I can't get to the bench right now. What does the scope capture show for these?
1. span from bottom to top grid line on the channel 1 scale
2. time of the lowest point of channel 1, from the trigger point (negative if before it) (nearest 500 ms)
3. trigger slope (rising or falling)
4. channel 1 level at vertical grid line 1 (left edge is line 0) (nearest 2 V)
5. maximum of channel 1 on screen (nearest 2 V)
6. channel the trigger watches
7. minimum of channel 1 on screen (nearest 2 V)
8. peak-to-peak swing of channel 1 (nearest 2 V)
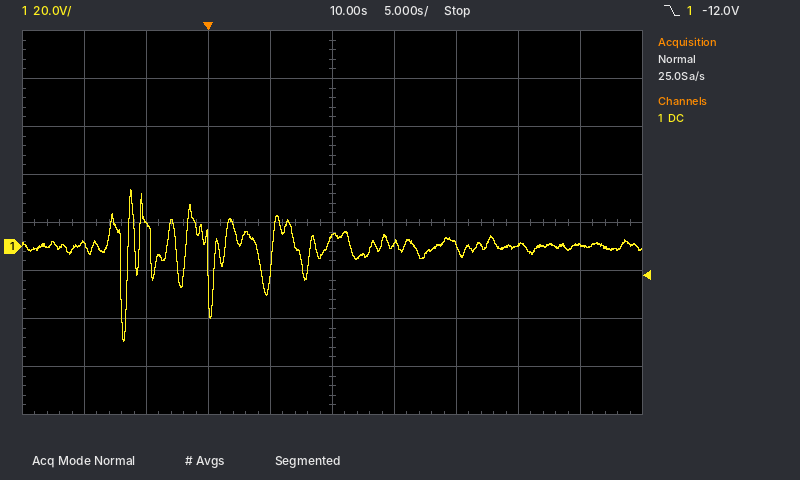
160 V
-7.0 s
falling
0 V
24 V
channel 1
-40 V
64 V
